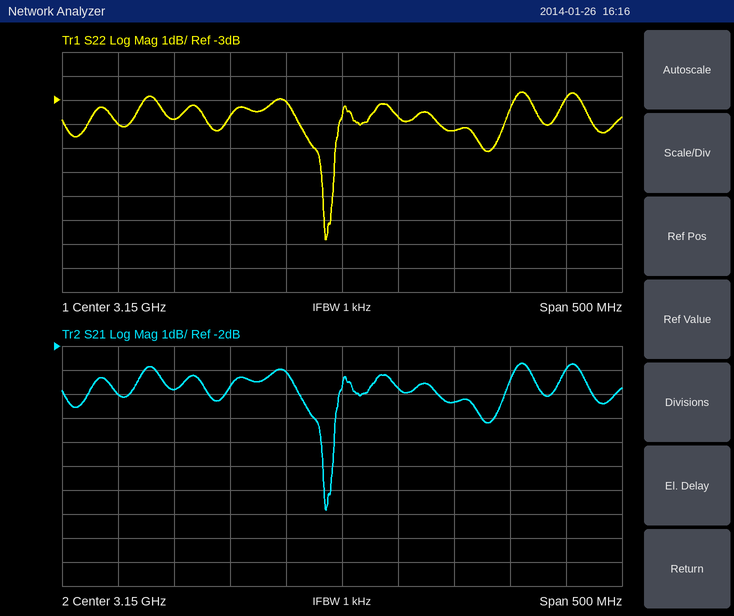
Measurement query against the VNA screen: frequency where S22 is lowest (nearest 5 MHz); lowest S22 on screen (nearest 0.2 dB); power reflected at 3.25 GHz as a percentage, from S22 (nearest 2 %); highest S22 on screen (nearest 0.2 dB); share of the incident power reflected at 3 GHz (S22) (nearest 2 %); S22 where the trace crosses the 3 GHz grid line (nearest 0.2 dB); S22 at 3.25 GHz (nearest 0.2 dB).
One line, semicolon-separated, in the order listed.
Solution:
3.135 GHz; -8.8 dB; 38 %; -2.6 dB; 42 %; -3.8 dB; -4.2 dB
